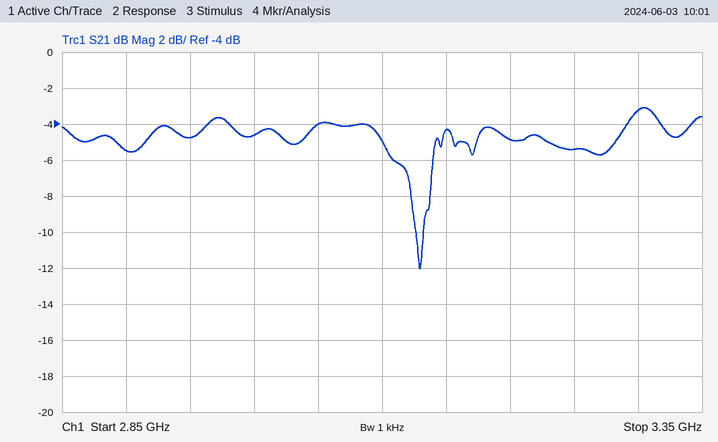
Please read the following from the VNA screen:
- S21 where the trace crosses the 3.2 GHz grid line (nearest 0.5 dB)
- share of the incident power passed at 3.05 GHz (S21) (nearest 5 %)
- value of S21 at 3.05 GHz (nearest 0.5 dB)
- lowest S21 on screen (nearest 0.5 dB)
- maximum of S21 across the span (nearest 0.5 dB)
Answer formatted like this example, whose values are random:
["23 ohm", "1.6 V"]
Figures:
["-5.0 dB", "40 %", "-4.0 dB", "-12.0 dB", "-3.0 dB"]
